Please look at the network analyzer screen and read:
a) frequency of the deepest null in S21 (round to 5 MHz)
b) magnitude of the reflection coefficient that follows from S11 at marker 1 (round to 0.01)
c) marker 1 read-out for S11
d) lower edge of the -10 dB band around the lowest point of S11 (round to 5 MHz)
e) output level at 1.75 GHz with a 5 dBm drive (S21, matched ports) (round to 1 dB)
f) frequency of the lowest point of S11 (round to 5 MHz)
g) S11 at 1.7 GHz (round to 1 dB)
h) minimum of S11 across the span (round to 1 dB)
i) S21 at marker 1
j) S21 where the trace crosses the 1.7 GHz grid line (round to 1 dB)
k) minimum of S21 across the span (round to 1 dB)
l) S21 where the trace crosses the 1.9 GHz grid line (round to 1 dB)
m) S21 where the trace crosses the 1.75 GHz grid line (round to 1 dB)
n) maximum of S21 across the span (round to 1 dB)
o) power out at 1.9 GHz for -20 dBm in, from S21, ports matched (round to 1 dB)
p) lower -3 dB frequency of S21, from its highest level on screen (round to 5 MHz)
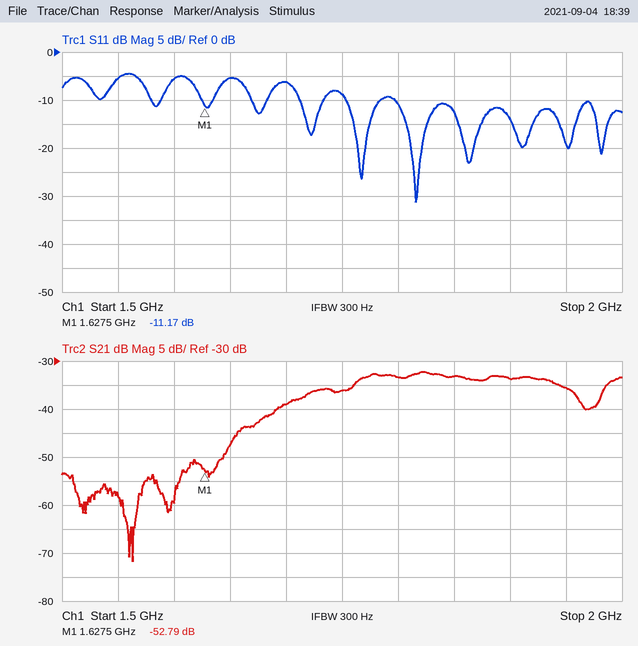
1.565 GHz
0.28
-11.17 dB
1.795 GHz
-31 dBm
1.815 GHz
-6 dB
-31 dB
-52.79 dB
-39 dB
-72 dB
-34 dB
-36 dB
-32 dB
-54 dBm
1.760 GHz
